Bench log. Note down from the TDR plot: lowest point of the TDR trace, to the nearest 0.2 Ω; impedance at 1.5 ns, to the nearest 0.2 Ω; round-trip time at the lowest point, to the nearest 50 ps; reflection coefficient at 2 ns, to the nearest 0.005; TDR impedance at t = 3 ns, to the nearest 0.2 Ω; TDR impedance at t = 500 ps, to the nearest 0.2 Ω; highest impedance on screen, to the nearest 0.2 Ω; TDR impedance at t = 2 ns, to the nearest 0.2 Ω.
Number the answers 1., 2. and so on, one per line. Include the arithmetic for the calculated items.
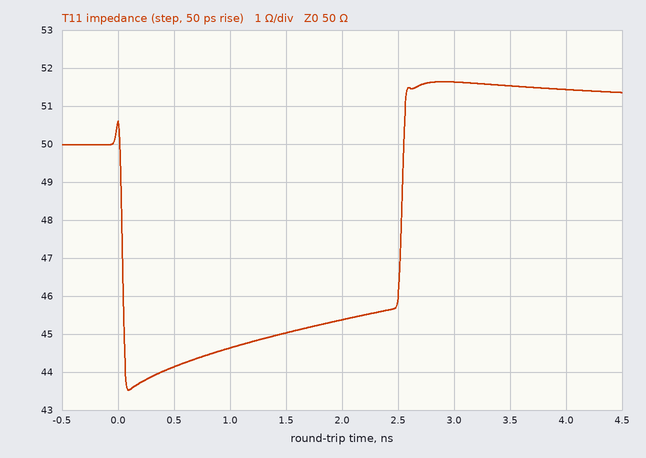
1. 43.6 Ω
2. 45.0 Ω
3. 100 ps
4. (45.4 − 50)/(45.4 + 50) ≈ -0.0482, so -0.050 to the nearest 0.005
5. 51.6 Ω
6. 44.2 Ω
7. 51.6 Ω
8. 45.4 Ω
